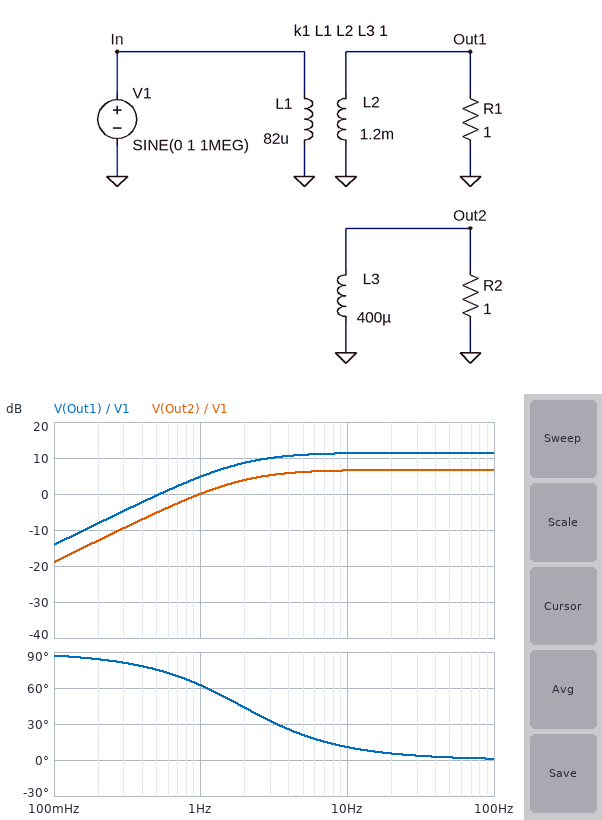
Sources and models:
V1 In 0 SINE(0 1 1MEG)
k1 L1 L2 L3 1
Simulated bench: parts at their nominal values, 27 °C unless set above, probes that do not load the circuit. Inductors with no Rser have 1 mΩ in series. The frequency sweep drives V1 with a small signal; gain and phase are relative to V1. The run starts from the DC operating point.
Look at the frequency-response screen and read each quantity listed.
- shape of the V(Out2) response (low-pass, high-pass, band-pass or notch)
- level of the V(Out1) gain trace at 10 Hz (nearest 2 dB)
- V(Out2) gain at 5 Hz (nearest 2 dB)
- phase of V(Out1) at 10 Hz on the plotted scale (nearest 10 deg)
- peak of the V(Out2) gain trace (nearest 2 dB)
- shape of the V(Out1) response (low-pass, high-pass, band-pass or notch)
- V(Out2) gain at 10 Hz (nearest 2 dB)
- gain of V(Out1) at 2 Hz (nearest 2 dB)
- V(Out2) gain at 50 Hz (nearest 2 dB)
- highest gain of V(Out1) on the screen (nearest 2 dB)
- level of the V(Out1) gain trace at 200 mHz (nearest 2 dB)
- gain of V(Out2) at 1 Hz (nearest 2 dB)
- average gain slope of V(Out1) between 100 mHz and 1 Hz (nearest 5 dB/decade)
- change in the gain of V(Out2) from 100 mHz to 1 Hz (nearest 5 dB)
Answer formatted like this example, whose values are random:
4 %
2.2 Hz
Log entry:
high-pass
12 dB
6 dB
10 deg
6 dB
high-pass
6 dB
8 dB
6 dB
12 dB
-8 dB
0 dB
20 dB/decade
20 dB
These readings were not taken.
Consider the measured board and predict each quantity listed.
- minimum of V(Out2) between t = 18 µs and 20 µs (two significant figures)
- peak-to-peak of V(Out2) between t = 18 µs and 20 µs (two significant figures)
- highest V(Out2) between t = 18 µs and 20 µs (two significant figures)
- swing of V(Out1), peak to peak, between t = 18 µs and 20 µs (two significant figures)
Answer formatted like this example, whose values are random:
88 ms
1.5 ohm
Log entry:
-2.2 V
4.3 V
2.2 V
7.5 V
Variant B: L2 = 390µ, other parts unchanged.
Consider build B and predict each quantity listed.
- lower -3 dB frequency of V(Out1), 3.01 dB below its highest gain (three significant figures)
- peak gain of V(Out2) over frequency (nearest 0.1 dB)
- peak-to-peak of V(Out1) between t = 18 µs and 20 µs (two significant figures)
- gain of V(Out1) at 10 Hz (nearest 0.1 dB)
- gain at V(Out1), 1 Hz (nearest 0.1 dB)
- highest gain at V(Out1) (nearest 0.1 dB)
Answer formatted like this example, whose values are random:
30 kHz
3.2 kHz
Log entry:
1.92 Hz
6.8 dB
4.3 V
6.5 dB
0 dB
6.7 dB
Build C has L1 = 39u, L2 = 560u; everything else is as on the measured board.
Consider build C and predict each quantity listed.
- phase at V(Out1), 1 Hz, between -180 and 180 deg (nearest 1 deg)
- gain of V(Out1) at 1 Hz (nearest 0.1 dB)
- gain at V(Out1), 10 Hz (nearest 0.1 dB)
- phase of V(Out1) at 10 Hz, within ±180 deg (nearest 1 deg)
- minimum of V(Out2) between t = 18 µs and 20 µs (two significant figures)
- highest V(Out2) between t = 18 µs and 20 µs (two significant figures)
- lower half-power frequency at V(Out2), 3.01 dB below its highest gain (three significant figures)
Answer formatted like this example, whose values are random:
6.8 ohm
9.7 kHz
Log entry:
76 deg
-0.9 dB
10.7 dB
22 deg
-3.1 V
3.1 V
3.98 Hz
